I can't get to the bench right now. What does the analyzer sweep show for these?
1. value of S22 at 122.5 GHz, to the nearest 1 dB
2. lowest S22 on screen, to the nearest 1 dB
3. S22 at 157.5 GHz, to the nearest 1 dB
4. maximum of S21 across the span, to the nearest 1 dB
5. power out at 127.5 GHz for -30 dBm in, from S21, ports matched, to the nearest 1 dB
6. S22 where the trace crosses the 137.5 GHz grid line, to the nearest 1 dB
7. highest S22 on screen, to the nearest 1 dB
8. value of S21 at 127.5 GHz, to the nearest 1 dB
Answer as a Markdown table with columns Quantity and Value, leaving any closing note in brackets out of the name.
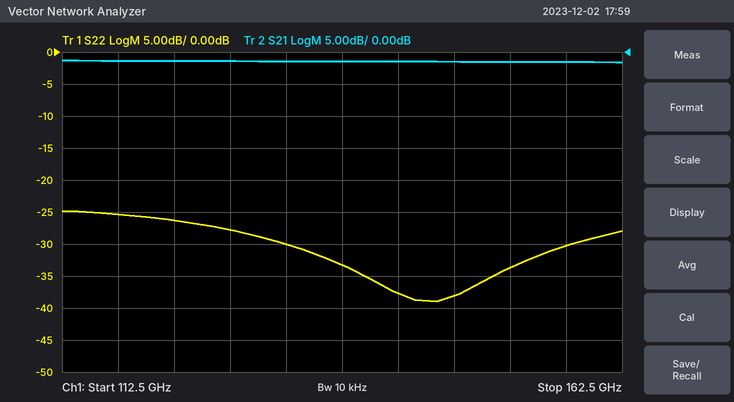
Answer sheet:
| Quantity | Value |
|---|---|
| value of S22 at 122.5 GHz, to the nearest 1 dB | -26 dB |
| lowest S22 on screen, to the nearest 1 dB | -39 dB |
| S22 at 157.5 GHz, to the nearest 1 dB | -30 dB |
| maximum of S21 across the span, to the nearest 1 dB | -1 dB |
| power out at 127.5 GHz for -30 dBm in, from S21, ports matched, to the nearest 1 dB | -31 dBm |
| S22 where the trace crosses the 137.5 GHz grid line, to the nearest 1 dB | -33 dB |
| highest S22 on screen, to the nearest 1 dB | -25 dB |
| value of S21 at 127.5 GHz, to the nearest 1 dB | -1 dB |
